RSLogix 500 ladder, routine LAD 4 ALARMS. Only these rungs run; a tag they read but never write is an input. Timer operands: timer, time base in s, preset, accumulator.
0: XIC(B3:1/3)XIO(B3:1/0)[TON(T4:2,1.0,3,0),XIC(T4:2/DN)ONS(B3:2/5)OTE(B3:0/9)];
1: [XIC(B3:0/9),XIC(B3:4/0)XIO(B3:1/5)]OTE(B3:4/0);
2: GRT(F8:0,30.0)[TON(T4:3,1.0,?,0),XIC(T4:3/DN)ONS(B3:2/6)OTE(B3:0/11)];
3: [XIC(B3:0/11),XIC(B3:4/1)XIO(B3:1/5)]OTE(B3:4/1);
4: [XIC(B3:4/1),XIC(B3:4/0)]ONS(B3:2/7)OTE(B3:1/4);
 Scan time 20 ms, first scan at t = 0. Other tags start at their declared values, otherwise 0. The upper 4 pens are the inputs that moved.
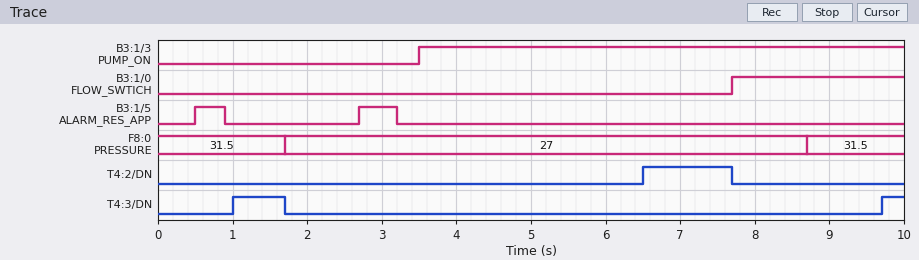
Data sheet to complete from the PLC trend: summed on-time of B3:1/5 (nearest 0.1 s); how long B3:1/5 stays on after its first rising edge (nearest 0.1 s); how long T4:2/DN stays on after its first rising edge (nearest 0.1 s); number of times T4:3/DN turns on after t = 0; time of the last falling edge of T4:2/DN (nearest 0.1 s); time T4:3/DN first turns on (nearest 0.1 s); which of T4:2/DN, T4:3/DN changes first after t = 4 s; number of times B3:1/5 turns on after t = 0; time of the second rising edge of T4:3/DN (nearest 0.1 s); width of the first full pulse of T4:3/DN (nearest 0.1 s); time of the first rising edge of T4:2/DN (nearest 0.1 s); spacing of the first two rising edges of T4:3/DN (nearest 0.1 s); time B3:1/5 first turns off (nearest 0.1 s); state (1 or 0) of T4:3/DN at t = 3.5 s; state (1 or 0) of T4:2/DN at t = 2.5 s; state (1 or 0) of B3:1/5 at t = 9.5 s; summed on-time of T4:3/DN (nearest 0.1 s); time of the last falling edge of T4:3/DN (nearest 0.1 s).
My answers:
0.9 s
0.4 s
1.2 s
2
7.7 s
1.0 s
T4:2/DN
2
9.7 s
0.7 s
6.5 s
8.7 s
0.9 s
0
0
0
1.0 s
1.7 s
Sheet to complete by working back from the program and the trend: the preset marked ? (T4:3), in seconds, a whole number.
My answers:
1 s
